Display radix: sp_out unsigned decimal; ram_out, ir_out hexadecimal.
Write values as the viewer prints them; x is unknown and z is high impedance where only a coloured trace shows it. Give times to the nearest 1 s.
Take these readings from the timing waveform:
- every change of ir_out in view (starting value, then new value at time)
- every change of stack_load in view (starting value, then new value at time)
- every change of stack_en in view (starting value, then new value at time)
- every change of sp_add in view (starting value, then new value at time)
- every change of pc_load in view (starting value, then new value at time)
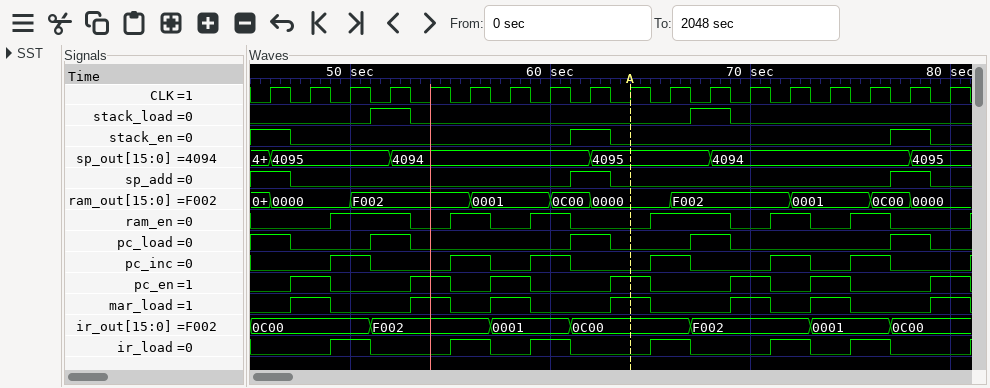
0C00, F002 at 51 s, 0001 at 57 s, 0C00 at 61 s, F002 at 67 s, 0001 at 73 s, 0C00 at 77 s
0, 1 at 51 s, 0 at 53 s, 1 at 67 s, 0 at 69 s
1, 0 at 47 s, 1 at 61 s, 0 at 63 s, 1 at 77 s, 0 at 79 s
1, 0 at 47 s, 1 at 61 s, 0 at 63 s, 1 at 77 s, 0 at 79 s
1, 0 at 47 s, 1 at 51 s, 0 at 53 s, 1 at 61 s, 0 at 63 s, 1 at 67 s, 0 at 69 s, 1 at 77 s, 0 at 79 s
